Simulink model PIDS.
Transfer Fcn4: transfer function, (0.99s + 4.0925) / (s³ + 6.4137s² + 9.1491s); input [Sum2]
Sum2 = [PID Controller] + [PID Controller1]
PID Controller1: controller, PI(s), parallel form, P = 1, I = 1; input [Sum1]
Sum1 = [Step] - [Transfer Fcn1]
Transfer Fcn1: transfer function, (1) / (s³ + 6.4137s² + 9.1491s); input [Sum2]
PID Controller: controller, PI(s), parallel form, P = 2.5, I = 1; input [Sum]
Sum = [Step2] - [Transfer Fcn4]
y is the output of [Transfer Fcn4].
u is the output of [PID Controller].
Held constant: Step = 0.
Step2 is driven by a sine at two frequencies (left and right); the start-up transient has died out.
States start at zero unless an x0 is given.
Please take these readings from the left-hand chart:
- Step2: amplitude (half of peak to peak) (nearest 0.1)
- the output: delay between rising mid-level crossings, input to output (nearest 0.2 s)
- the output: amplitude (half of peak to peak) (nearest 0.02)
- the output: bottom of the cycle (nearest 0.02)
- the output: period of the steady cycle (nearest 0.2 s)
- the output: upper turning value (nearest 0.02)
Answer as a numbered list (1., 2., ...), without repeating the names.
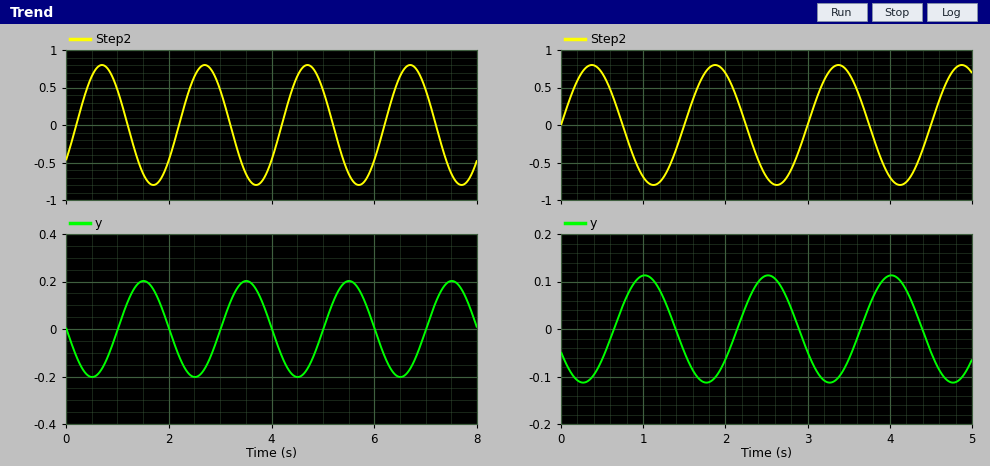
1. 0.8
2. 0.8 s
3. 0.20
4. -0.20
5. 2.0 s
6. 0.20
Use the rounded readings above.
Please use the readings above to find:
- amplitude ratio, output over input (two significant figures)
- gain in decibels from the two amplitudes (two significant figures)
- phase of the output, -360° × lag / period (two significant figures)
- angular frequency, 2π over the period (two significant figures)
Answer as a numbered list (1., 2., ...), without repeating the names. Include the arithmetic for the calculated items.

1. 0.2 / 0.8 = 0.25
2. 20 log10(0.2 / 0.8) = -12 dB
3. -360 × 0.8 / 2 = -140°
4. 2π / 2 = 3.1 rad/s
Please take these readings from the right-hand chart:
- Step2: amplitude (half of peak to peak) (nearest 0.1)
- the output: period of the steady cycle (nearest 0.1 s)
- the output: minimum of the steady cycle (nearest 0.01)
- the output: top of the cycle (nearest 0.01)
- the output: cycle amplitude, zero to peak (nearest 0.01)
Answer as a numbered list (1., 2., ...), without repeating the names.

1. 0.8
2. 1.5 s
3. -0.11
4. 0.11
5. 0.11
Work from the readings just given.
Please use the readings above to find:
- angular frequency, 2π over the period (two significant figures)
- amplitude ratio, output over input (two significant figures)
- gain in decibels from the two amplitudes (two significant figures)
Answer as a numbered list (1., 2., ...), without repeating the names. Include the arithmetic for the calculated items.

1. 2π / 1.5 = 4.2 rad/s
2. 0.11 / 0.8 = 0.14
3. 20 log10(0.11 / 0.8) = -17 dB
